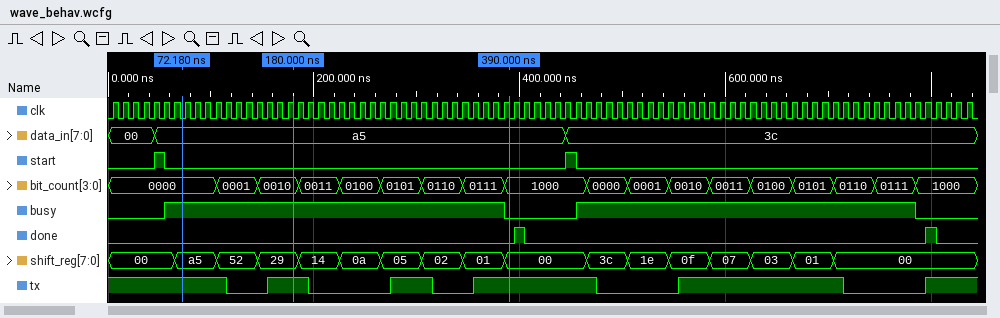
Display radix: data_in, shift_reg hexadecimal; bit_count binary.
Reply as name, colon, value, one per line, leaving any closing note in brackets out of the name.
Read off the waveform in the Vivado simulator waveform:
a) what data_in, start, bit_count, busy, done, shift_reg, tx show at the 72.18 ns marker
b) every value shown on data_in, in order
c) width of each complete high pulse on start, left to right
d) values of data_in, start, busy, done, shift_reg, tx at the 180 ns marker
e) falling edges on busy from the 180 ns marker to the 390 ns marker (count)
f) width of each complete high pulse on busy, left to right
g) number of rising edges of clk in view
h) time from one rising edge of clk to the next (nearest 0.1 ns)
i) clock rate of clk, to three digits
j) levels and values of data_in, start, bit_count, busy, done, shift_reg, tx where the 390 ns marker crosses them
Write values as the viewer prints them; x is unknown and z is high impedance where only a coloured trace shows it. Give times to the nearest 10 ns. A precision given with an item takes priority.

what data_in, start, bit_count, busy, done, shift_reg, tx show at the 72.18 ns marker: data_in=a5, start=0, bit_count=0000, busy=1, done=0, shift_reg=a5, tx=1
every value shown on data_in, in order: 00, a5, 3c
width of each complete high pulse on start, left to right: 10 ns, 10 ns
values of data_in, start, busy, done, shift_reg, tx at the 180 ns marker: data_in=a5, start=0, busy=1, done=0, shift_reg=29, tx=1
falling edges on busy from the 180 ns marker to the 390 ns marker: 1
width of each complete high pulse on busy, left to right: 330 ns, 330 ns
number of rising edges of clk in view: 84
time from one rising edge of clk to the next: 10 ns
clock rate of clk, to three digits: 100 MHz
levels and values of data_in, start, bit_count, busy, done, shift_reg, tx where the 390 ns marker crosses them: data_in=a5, start=0, bit_count=1000, busy=0, done=0, shift_reg=00, tx=1
